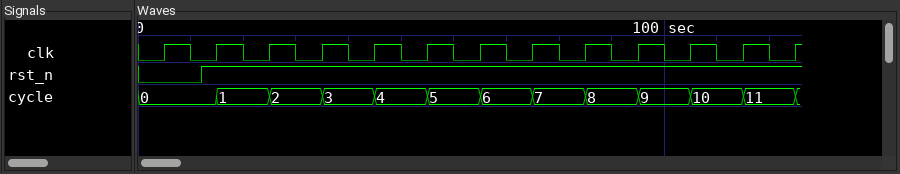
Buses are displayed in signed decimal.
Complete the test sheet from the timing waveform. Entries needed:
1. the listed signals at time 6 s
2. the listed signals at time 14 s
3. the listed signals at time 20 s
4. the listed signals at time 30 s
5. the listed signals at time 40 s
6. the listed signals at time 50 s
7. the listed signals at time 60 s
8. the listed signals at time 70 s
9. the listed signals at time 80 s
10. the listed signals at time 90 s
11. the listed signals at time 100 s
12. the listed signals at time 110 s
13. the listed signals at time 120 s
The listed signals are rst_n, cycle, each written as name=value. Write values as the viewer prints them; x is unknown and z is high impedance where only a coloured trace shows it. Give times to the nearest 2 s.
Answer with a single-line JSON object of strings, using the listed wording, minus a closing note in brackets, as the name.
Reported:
{"the listed signals at time 6 s": "rst_n=0, cycle=0", "the listed signals at time 14 s": "rst_n=1, cycle=0", "the listed signals at time 20 s": "rst_n=1, cycle=1", "the listed signals at time 30 s": "rst_n=1, cycle=2", "the listed signals at time 40 s": "rst_n=1, cycle=3", "the listed signals at time 50 s": "rst_n=1, cycle=4", "the listed signals at time 60 s": "rst_n=1, cycle=5", "the listed signals at time 70 s": "rst_n=1, cycle=6", "the listed signals at time 80 s": "rst_n=1, cycle=7", "the listed signals at time 90 s": "rst_n=1, cycle=8", "the listed signals at time 100 s": "rst_n=1, cycle=9", "the listed signals at time 110 s": "rst_n=1, cycle=10", "the listed signals at time 120 s": "rst_n=1, cycle=11"}
